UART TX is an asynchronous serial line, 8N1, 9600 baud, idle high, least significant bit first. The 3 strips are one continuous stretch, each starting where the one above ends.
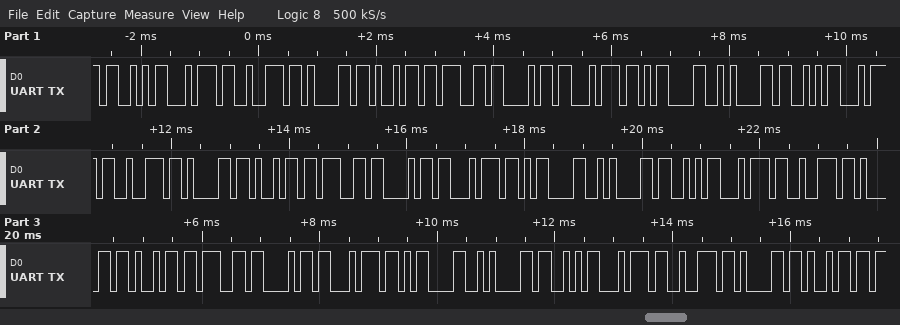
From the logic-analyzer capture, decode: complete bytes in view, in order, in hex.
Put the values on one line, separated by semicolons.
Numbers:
53 74 72 61 69 67 68 74 0D 0A 53 74 72 61 69 67 68 74 0D 0A 53 74 72 61 69 67 68 74 0D 0A 53 74 72 61 69
